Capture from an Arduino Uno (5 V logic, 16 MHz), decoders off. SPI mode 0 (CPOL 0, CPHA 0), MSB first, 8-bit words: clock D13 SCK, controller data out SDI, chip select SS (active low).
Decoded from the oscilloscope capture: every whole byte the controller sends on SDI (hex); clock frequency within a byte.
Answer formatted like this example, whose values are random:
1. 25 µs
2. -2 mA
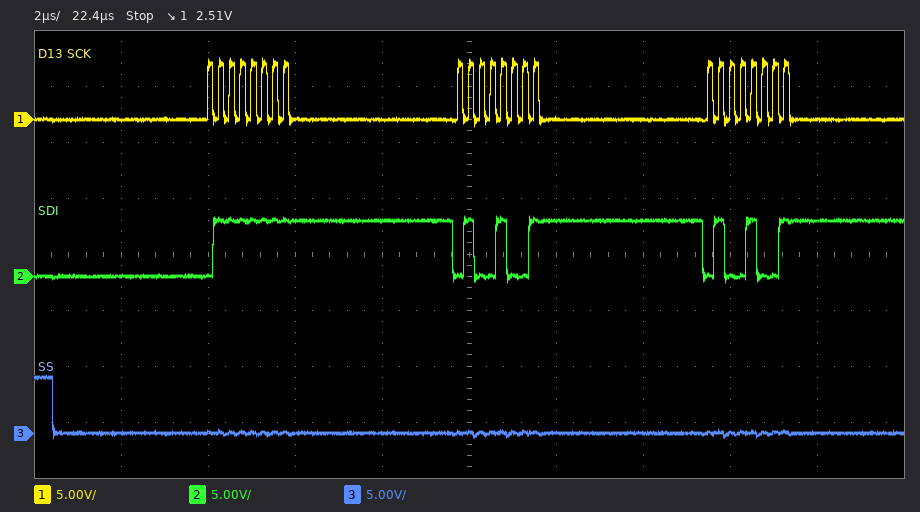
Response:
1. 7F 49 49
2. 4 MHz
